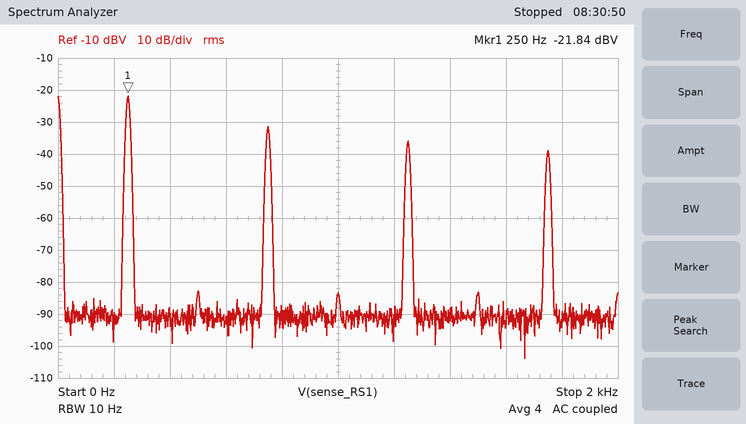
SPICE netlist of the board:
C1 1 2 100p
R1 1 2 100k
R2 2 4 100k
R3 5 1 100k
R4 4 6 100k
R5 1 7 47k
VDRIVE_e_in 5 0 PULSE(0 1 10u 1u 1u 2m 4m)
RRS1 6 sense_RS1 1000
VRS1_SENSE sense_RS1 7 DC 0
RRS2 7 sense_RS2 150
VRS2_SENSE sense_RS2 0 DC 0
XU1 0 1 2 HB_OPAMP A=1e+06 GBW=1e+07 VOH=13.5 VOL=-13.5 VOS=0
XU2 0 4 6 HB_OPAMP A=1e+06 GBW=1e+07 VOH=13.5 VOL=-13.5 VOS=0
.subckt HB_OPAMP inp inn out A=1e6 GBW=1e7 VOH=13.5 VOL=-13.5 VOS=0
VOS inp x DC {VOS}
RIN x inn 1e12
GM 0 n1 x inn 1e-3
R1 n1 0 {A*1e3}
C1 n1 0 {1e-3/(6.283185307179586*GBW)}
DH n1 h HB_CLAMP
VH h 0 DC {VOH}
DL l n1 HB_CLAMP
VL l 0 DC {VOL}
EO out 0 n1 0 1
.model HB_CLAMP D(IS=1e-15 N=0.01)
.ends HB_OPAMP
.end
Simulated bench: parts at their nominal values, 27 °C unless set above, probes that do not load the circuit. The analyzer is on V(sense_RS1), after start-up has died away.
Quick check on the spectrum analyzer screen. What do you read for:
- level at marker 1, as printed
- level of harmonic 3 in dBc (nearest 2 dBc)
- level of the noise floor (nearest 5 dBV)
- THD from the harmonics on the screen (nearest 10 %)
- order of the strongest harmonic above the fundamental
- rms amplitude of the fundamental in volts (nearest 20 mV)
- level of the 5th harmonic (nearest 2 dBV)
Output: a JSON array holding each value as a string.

["-21.84 dBV", "-10 dBc", "-90 dBV", "40 %", "3", "80 mV", "-36 dBV"]
